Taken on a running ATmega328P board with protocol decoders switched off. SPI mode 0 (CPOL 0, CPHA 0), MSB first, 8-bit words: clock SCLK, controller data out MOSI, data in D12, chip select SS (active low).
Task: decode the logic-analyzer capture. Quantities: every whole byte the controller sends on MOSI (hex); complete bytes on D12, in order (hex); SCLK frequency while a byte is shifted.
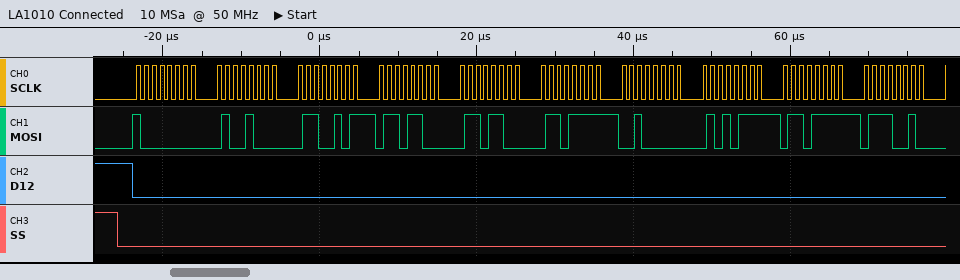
80 48 65 6C 6C 6F 20 57 6F 72
00 00 00 00 00 00 00 00 00 00
1 MHz
